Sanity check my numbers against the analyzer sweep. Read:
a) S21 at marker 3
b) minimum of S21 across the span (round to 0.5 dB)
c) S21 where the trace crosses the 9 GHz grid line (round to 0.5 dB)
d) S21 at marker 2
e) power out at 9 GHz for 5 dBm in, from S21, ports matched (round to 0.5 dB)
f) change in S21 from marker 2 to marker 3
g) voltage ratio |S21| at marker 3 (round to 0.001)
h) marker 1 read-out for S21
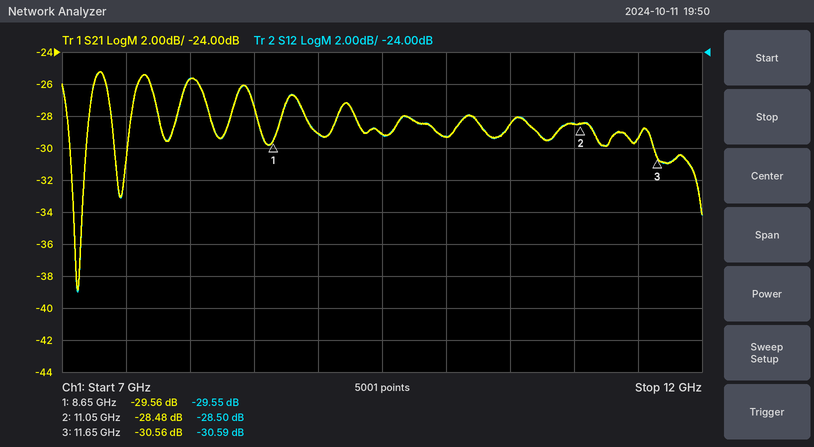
-30.56 dB
-39.0 dB
-29.0 dB
-28.48 dB
-24.0 dBm
-2.08 dB
0.030
-29.56 dB
